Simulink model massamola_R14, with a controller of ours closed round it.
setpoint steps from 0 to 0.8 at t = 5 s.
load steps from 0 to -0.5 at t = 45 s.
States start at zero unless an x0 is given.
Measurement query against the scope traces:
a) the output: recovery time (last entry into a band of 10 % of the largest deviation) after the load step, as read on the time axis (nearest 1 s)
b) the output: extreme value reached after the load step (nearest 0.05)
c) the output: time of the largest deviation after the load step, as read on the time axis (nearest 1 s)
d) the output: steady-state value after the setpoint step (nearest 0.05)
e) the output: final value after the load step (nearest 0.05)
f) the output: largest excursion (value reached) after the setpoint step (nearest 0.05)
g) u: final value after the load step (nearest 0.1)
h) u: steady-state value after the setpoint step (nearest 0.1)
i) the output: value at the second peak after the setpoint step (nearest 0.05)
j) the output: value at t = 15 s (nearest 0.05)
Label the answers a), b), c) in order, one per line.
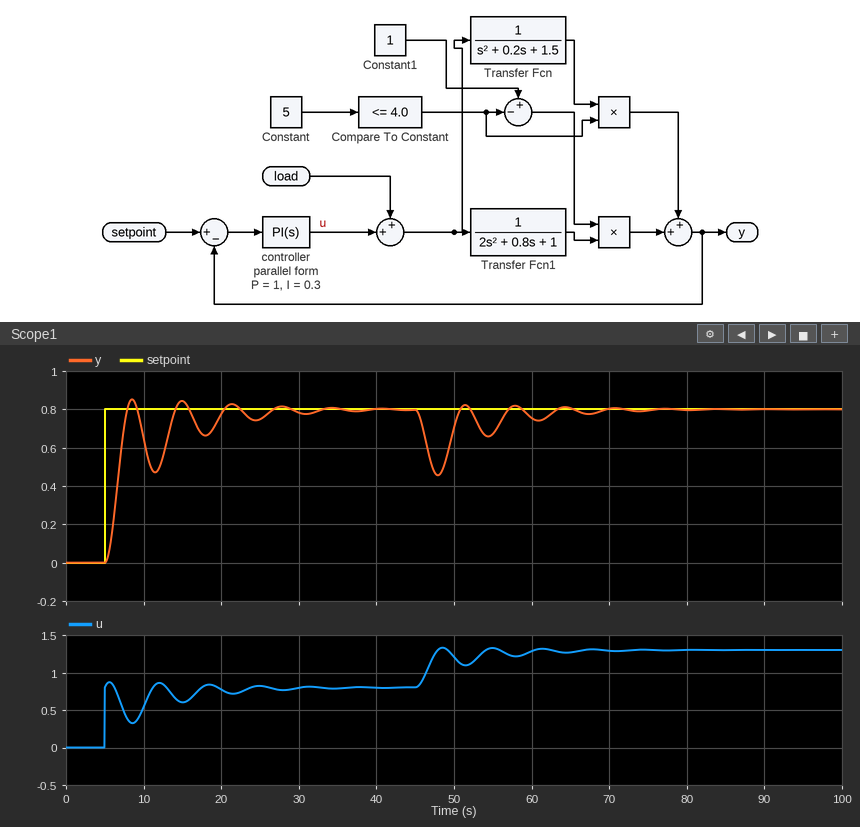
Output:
a) 62 s
b) 0.45
c) 48 s
d) 0.80
e) 0.80
f) 0.85
g) 1.3
h) 0.8
i) 0.85
j) 0.85
